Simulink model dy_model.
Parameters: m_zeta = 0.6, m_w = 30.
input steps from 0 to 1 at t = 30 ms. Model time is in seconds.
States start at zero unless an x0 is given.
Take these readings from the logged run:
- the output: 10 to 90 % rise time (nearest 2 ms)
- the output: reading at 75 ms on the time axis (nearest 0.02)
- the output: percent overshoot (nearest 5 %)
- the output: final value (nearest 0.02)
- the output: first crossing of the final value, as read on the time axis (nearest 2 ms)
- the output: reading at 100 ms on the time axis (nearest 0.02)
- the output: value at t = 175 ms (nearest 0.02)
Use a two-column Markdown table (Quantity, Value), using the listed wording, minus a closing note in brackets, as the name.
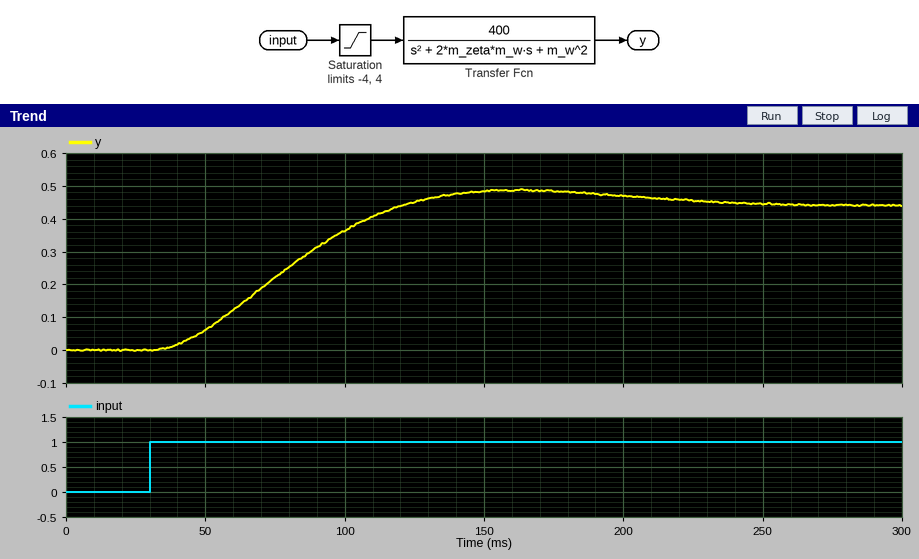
| Quantity | Value |
|---|---|
| the output: 10 to 90 % rise time | 62 ms |
| the output: reading at 75 ms on the time axis | 0.22 |
| the output: percent overshoot | 10 % |
| the output: final value | 0.44 |
| the output: first crossing of the final value, as read on the time axis | 122 ms |
| the output: reading at 100 ms on the time axis | 0.36 |
| the output: value at t = 175 ms | 0.48 |
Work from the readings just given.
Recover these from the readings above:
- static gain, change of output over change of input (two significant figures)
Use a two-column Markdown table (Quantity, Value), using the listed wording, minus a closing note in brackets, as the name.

| Quantity | Value |
|---|---|
| static gain, change of output over change of input | 0.44 |
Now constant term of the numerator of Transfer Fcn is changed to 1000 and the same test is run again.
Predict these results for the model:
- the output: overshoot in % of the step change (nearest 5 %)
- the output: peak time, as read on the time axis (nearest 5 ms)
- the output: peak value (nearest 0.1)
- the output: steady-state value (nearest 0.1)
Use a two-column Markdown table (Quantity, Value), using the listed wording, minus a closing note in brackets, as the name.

| Quantity | Value |
|---|---|
| the output: overshoot in % of the step change | 10 % |
| the output: peak time, as read on the time axis | 160 ms |
| the output: peak value | 1.2 |
| the output: steady-state value | 1.1 |
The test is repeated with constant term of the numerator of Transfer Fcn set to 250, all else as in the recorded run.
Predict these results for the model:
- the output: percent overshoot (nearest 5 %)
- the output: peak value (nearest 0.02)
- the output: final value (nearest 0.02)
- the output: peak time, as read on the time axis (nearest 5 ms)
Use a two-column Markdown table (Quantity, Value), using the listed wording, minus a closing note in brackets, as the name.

| Quantity | Value |
|---|---|
| the output: percent overshoot | 10 % |
| the output: peak value | 0.30 |
| the output: final value | 0.28 |
| the output: peak time, as read on the time axis | 160 ms |
